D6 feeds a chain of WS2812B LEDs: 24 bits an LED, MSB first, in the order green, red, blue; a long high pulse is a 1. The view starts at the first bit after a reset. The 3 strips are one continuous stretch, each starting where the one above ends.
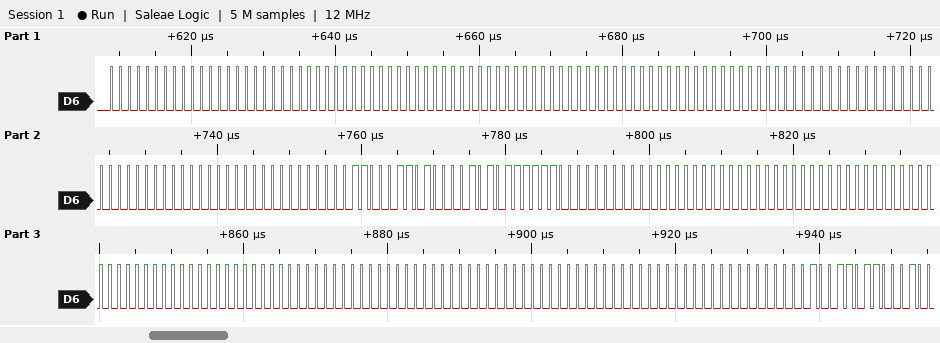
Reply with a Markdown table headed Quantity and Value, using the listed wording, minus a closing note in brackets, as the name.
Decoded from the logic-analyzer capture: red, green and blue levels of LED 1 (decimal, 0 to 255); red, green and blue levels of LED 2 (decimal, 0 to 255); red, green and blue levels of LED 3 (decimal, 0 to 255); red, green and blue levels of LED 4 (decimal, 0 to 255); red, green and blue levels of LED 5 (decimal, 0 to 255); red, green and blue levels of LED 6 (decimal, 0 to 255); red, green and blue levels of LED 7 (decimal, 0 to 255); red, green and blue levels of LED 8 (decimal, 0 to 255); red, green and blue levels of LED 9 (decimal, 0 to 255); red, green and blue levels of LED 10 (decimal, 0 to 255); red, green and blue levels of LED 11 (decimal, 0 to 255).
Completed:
| Quantity | Value |
|---|---|
| red, green and blue levels of LED 1 | 0, 0, 0 |
| red, green and blue levels of LED 2 | 0, 0, 0 |
| red, green and blue levels of LED 3 | 0, 0, 0 |
| red, green and blue levels of LED 4 | 0, 0, 0 |
| red, green and blue levels of LED 5 | 0, 0, 0 |
| red, green and blue levels of LED 6 | 133, 198, 126 |
| red, green and blue levels of LED 7 | 0, 0, 0 |
| red, green and blue levels of LED 8 | 0, 0, 0 |
| red, green and blue levels of LED 9 | 0, 0, 0 |
| red, green and blue levels of LED 10 | 0, 0, 0 |
| red, green and blue levels of LED 11 | 0, 0, 0 |
